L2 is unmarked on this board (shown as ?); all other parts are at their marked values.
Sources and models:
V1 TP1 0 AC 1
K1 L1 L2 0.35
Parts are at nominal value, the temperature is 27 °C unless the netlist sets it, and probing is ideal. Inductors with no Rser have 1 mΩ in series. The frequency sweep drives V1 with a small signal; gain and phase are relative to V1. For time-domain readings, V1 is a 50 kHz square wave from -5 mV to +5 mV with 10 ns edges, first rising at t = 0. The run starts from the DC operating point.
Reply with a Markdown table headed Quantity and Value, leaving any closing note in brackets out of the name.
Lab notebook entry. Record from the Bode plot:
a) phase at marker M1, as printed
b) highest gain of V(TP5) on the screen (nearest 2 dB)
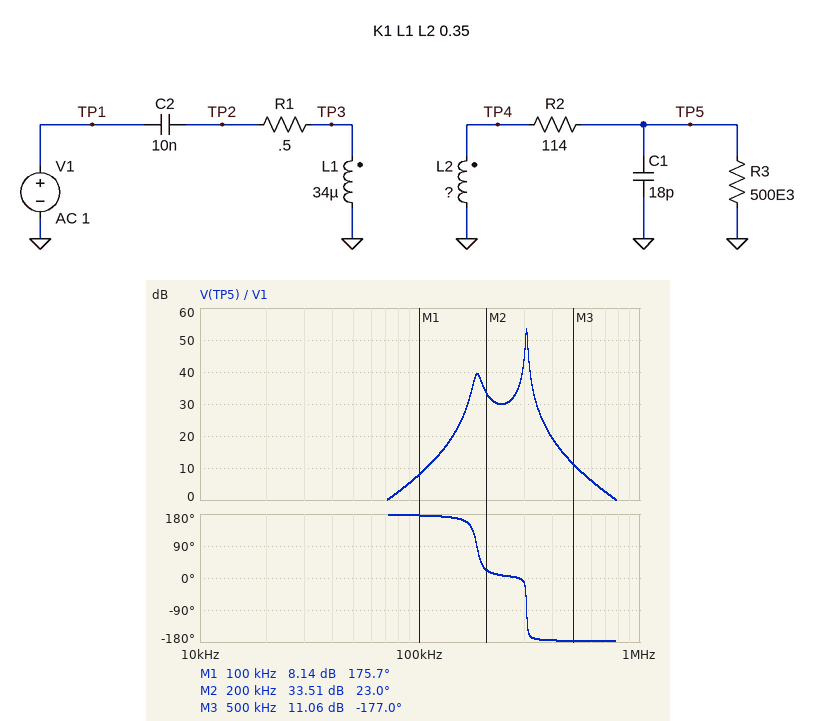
| Quantity | Value |
|---|---|
| phase at marker M1, as printed | 175.7 deg |
| highest gain of V(TP5) on the screen | 54 dB |
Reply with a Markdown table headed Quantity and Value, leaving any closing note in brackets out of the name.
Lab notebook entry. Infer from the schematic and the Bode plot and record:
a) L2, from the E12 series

| Quantity | Value |
|---|---|
| L2, from the E12 series | 39 mH |
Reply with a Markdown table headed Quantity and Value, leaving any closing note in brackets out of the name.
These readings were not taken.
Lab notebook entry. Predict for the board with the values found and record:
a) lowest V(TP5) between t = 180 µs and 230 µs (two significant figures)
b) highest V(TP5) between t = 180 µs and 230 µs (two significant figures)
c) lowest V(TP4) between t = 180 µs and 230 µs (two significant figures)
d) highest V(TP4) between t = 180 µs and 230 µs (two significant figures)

| Quantity | Value |
|---|---|
| lowest V(TP5) between t = 180 µs and 230 µs | -86 mV |
| highest V(TP5) between t = 180 µs and 230 µs | 89 mV |
| lowest V(TP4) between t = 180 µs and 230 µs | -86 mV |
| highest V(TP4) between t = 180 µs and 230 µs | 89 mV |
